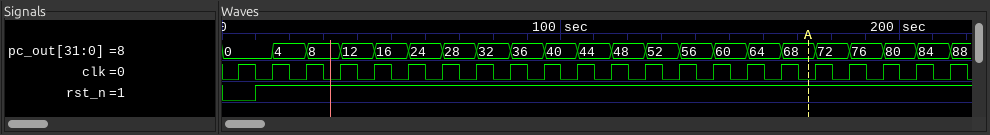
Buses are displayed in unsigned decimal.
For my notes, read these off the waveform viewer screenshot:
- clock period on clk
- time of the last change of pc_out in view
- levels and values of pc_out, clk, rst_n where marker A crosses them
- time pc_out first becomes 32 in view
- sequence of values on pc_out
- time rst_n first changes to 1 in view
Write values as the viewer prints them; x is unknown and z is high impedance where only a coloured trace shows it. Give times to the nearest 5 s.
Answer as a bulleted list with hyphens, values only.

- 10 s
- 215 s
- pc_out=68, clk=0, rst_n=1
- 75 s
- 0, 4, 8, 12, 16, 24, 28, 32, 36, 40, 44, 48, 52, 56, 60, 64, 68, 72, 76, 80, 84, 88
- 10 s
